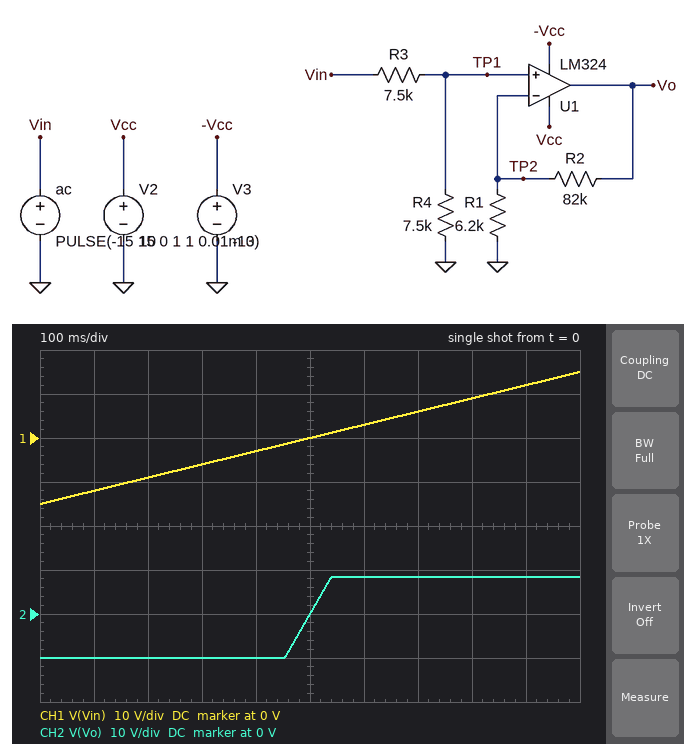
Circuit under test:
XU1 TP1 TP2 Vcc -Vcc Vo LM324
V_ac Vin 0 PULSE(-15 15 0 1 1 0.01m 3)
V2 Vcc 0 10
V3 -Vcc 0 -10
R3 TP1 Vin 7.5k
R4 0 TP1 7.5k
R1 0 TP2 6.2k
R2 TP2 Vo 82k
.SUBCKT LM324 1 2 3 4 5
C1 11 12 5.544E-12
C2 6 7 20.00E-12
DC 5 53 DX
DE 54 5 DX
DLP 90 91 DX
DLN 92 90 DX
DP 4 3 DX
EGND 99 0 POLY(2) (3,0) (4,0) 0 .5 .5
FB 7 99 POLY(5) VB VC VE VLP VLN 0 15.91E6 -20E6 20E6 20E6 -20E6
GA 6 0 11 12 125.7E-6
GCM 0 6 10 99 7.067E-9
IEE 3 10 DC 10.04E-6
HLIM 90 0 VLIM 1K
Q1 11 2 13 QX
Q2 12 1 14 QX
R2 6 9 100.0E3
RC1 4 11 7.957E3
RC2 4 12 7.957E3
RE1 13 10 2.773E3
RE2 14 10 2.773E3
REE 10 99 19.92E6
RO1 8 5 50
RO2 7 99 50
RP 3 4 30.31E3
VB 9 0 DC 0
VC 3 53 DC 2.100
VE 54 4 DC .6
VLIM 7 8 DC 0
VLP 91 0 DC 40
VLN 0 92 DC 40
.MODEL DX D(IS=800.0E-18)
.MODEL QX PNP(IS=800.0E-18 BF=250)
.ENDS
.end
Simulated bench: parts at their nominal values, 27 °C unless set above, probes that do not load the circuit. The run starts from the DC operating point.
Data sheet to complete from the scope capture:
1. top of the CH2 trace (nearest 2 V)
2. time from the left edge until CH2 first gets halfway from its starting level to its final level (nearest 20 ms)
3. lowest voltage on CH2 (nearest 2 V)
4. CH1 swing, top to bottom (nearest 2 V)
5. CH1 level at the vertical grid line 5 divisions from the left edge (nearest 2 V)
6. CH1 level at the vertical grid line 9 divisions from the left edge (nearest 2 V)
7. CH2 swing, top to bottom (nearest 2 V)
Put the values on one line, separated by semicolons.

8 V; 500 ms; -10 V; 30 V; 0 V; 12 V; 18 V
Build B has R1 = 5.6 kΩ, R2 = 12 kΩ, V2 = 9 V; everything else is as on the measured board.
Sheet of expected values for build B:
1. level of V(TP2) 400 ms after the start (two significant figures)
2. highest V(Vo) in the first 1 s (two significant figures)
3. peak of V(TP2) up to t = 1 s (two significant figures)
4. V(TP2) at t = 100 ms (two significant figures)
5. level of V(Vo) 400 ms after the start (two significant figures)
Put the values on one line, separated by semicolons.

-1.5 V; 7.5 V; 2.4 V; -3.2 V; -4.7 V
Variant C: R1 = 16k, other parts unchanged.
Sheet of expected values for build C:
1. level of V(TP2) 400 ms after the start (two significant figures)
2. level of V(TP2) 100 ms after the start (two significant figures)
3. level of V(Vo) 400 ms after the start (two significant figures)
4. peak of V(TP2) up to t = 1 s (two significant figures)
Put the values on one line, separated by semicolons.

-1.5 V; -1.6 V; -9.2 V; 1.4 V
